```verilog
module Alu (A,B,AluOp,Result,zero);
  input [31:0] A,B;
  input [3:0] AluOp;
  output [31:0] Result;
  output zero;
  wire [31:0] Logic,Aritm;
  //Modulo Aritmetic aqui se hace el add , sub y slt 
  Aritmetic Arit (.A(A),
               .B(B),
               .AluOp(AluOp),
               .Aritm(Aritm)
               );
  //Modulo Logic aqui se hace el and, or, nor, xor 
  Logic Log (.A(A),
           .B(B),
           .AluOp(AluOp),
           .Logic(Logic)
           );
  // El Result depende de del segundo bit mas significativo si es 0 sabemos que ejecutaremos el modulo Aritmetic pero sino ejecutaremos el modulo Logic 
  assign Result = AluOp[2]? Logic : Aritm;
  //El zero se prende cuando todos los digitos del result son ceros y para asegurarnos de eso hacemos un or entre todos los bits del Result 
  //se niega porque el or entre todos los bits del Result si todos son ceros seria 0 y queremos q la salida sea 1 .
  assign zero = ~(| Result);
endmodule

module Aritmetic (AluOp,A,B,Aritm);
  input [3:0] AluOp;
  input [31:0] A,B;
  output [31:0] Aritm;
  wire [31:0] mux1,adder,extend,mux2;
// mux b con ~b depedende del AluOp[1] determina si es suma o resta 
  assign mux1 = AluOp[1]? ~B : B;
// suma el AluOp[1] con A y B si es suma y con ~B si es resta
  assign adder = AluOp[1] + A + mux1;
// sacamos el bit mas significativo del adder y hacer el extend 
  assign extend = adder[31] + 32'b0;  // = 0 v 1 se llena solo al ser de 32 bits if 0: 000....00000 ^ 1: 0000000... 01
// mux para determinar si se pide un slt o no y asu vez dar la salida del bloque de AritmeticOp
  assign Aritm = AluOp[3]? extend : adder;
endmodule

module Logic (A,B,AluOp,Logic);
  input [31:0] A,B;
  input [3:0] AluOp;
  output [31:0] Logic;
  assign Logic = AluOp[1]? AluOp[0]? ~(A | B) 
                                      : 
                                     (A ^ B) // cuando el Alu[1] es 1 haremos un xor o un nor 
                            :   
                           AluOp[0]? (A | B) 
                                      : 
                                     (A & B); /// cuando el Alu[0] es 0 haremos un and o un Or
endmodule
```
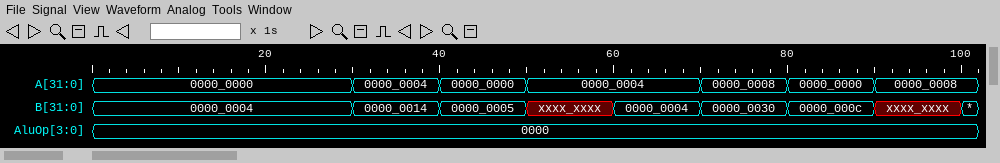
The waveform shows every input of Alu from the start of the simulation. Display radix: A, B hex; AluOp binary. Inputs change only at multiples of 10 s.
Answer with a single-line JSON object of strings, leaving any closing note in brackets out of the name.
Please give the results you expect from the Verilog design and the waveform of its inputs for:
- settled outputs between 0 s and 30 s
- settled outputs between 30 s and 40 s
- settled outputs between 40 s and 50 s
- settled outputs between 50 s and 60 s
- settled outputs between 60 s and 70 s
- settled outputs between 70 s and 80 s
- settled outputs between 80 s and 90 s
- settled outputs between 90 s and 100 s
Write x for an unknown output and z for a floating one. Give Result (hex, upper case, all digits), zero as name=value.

{"settled outputs between 0 s and 30 s": "Result=00000004, zero=0", "settled outputs between 30 s and 40 s": "Result=00000018, zero=0", "settled outputs between 40 s and 50 s": "Result=00000005, zero=0", "settled outputs between 50 s and 60 s": "Result=x, zero=x", "settled outputs between 60 s and 70 s": "Result=00000008, zero=0", "settled outputs between 70 s and 80 s": "Result=00000038, zero=0", "settled outputs between 80 s and 90 s": "Result=0000000C, zero=0", "settled outputs between 90 s and 100 s": "Result=x, zero=x"}
